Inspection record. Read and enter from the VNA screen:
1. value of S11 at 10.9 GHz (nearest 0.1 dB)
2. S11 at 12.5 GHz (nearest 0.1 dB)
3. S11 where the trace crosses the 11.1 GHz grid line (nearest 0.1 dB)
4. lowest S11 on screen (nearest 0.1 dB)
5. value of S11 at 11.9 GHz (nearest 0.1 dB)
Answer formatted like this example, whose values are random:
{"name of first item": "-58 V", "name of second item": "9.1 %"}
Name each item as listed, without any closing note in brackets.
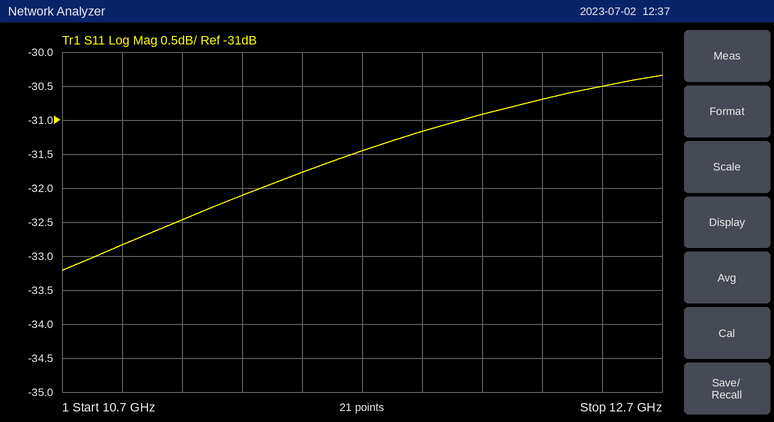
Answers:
{"value of S11 at 10.9 GHz": "-32.8 dB", "S11 at 12.5 GHz": "-30.5 dB", "S11 where the trace crosses the 11.1 GHz grid line": "-32.5 dB", "lowest S11 on screen": "-33.2 dB", "value of S11 at 11.9 GHz": "-31.2 dB"}
